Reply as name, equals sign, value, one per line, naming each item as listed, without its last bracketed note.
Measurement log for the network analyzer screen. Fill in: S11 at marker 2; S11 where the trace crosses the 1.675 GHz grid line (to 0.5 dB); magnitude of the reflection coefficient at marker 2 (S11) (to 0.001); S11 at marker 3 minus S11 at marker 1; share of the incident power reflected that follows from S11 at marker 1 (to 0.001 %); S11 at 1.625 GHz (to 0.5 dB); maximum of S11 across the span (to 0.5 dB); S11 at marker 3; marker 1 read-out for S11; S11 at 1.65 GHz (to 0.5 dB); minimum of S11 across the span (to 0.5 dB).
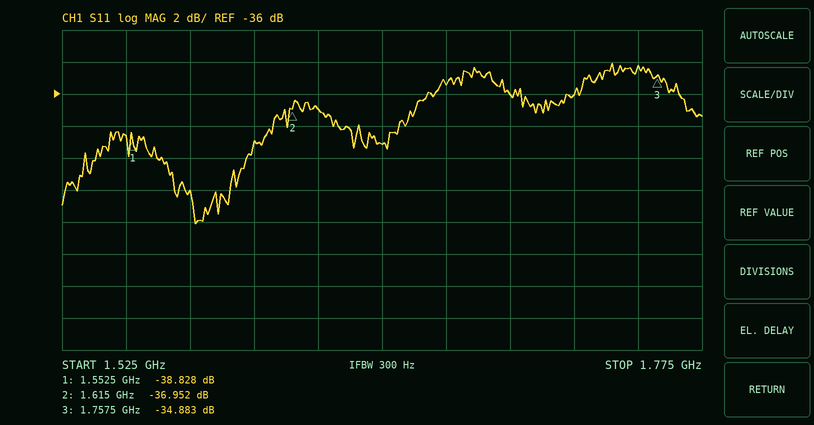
S11 at marker 2 = -36.952 dB
S11 where the trace crosses the 1.675 GHz grid line = -35.5 dB
magnitude of the reflection coefficient at marker 2 (S11) = 0.014
S11 at marker 3 minus S11 at marker 1 = 3.945 dB
share of the incident power reflected that follows from S11 at marker 1 = 0.013 %
S11 at 1.625 GHz = -37.0 dB
maximum of S11 across the span = -34.0 dB
S11 at marker 3 = -34.883 dB
marker 1 read-out for S11 = -38.828 dB
S11 at 1.65 GHz = -39.0 dB
minimum of S11 across the span = -44.0 dB
